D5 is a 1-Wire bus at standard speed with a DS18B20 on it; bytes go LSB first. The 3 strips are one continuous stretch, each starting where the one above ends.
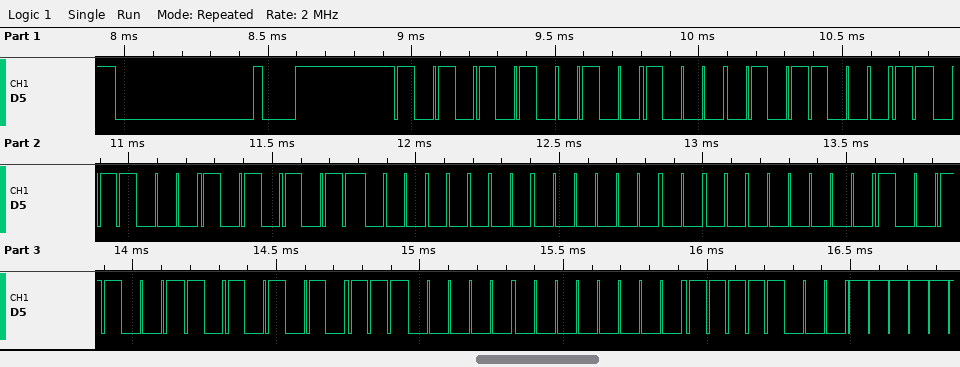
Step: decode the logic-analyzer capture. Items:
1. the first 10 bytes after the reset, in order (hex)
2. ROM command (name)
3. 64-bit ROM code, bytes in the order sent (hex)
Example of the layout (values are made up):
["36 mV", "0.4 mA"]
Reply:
["55 12 1A 1B D5 00 00 00 99 55", "Match ROM", "12 1A 1B D5 00 00 00 99"]
